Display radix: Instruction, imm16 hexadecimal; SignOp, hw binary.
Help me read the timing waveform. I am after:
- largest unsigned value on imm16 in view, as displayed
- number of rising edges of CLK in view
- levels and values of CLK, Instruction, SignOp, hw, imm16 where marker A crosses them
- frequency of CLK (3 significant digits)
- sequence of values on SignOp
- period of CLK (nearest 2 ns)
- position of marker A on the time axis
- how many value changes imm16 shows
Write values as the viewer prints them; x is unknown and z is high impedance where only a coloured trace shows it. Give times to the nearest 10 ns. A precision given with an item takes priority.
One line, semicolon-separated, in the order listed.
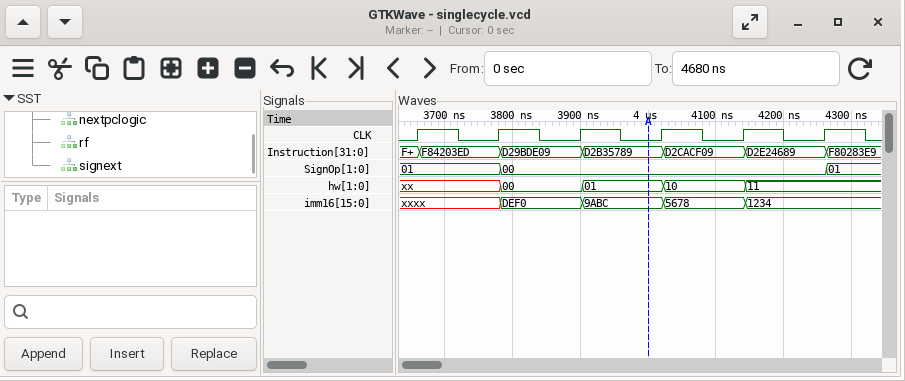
DEF0; 6; CLK=0, Instruction=D2B35789, SignOp=00, hw=01, imm16=9ABC; 8.33 MHz; 01, 00, 01; 120 ns; 4000 ns; 4
